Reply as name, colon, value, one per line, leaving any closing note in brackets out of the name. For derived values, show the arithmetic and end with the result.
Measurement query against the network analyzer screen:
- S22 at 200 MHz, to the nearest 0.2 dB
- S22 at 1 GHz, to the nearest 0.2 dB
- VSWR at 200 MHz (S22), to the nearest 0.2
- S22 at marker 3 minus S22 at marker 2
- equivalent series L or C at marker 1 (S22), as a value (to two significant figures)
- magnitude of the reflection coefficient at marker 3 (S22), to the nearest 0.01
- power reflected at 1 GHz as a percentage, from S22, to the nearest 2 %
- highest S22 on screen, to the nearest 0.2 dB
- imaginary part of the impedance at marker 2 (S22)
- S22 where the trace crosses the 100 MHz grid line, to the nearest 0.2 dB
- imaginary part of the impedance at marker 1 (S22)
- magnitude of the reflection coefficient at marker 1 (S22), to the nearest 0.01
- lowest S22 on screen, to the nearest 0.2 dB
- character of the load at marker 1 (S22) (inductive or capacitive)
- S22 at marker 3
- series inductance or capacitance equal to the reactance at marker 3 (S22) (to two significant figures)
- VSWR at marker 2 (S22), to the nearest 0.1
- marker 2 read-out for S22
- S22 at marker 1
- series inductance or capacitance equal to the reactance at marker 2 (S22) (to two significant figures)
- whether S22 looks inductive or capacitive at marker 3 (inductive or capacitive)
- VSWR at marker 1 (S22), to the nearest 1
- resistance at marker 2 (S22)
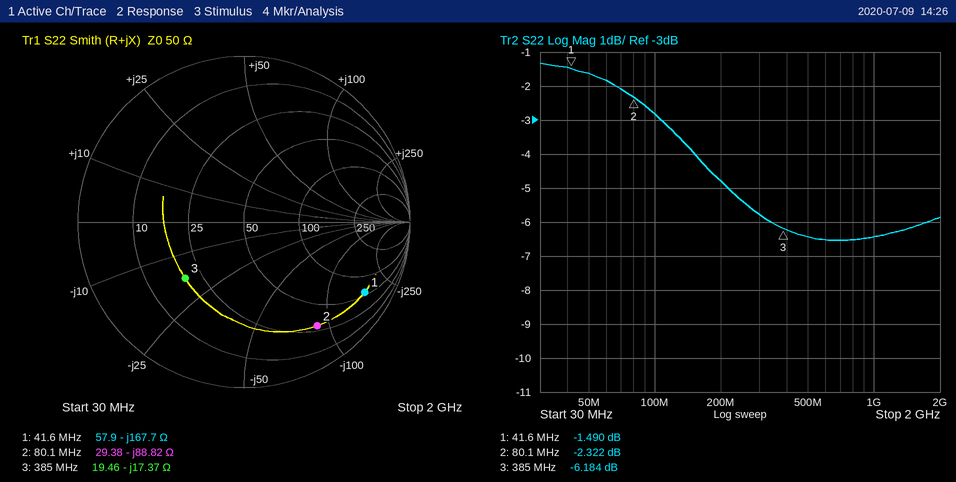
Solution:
S22 at 200 MHz, to the nearest 0.2 dB: -4.8 dB
S22 at 1 GHz, to the nearest 0.2 dB: -6.4 dB
VSWR at 200 MHz (S22), to the nearest 0.2: |Γ| = 10^(-4.8/20) = 0.5754; VSWR = (1 + 0.5754)/(1 − 0.5754) ≈ 3.71, so 3.8 to the nearest 0.2
S22 at marker 3 minus S22 at marker 2: -6.184 − (-2.322) = -3.862 dB
equivalent series L or C at marker 1 (S22), as a value: C = 1/(2π × 41.6 MHz × 167.7 Ω) ≈ 23 pF
magnitude of the reflection coefficient at marker 3 (S22), to the nearest 0.01: 0.49
power reflected at 1 GHz as a percentage, from S22, to the nearest 2 %: 10^(-6.4/10) ≈ 22.9 %, so 22 % to the nearest 2 %
highest S22 on screen, to the nearest 0.2 dB: -1.4 dB
imaginary part of the impedance at marker 2: -88.82 Ω
S22 where the trace crosses the 100 MHz grid line, to the nearest 0.2 dB: -2.8 dB
imaginary part of the impedance at marker 1: -167.7 Ω
magnitude of the reflection coefficient at marker 1 (S22), to the nearest 0.01: 0.84
lowest S22 on screen, to the nearest 0.2 dB: -6.6 dB
character of the load at marker 1 (S22): capacitive
S22 at marker 3: -6.184 dB
series inductance or capacitance equal to the reactance at marker 3 (S22): C = 1/(2π × 385 MHz × 17.37 Ω) ≈ 24 pF
VSWR at marker 2 (S22), to the nearest 0.1: 7.5
marker 2 read-out for S22: -2.322 dB
S22 at marker 1: -1.490 dB
series inductance or capacitance equal to the reactance at marker 2 (S22): C = 1/(2π × 80.1 MHz × 88.82 Ω) ≈ 22 pF
whether S22 looks inductive or capacitive at marker 3: capacitive
VSWR at marker 1 (S22), to the nearest 1: (1 + 0.8424)/(1 − 0.8424) ≈ 12
resistance at marker 2: 29.38 Ω
